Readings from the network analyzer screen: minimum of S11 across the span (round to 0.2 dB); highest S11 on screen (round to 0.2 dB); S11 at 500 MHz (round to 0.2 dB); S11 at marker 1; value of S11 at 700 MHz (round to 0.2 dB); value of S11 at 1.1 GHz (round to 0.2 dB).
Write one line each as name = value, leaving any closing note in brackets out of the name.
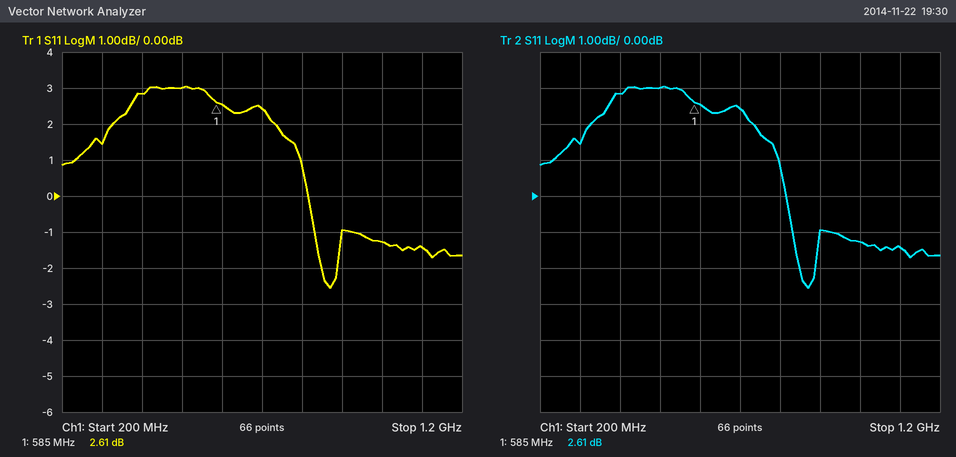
minimum of S11 across the span = -2.6 dB
highest S11 on screen = 3.0 dB
S11 at 500 MHz = 3.0 dB
S11 at marker 1 = 2.61 dB
value of S11 at 700 MHz = 2.4 dB
value of S11 at 1.1 GHz = -1.4 dB
